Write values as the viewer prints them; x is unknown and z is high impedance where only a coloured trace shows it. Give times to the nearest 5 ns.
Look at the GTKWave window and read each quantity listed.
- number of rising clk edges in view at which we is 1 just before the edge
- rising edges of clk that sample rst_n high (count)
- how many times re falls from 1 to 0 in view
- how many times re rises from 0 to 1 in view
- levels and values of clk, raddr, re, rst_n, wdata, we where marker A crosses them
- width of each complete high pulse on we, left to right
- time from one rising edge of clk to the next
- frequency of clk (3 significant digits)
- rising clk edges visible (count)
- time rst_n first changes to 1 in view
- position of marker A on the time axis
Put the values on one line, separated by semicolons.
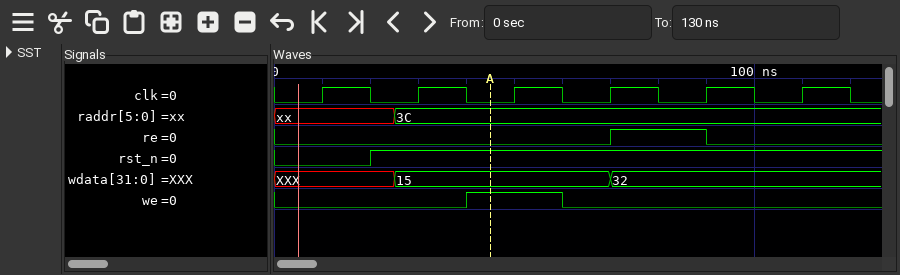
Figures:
1; 5; 1; 1; clk=0, raddr=3C, re=0, rst_n=1, wdata=15, we=1; 20 ns; 20 ns; 50.0 MHz; 6; 20 ns; 45 ns
